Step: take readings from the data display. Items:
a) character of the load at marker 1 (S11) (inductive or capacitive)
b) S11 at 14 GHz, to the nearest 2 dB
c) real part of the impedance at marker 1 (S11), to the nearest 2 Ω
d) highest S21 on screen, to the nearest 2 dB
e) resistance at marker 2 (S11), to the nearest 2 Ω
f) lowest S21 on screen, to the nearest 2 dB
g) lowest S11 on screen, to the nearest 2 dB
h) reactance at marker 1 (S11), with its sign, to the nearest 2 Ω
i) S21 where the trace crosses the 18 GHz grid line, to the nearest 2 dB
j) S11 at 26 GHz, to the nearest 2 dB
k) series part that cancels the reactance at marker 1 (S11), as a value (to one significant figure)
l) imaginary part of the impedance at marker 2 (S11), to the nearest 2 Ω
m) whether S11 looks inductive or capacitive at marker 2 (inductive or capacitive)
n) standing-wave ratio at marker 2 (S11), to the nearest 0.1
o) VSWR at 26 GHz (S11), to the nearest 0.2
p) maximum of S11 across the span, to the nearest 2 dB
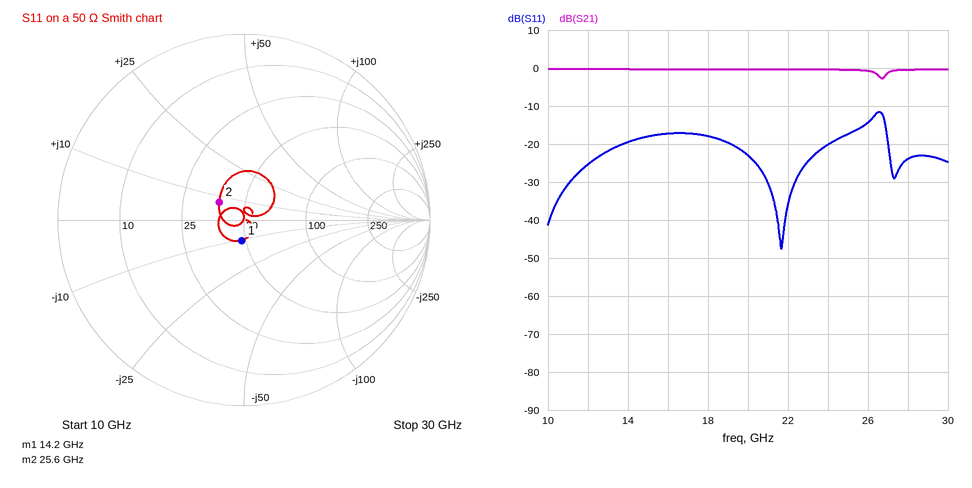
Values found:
capacitive
-20 dB
48 Ω
0 dB
38 Ω
-2 dB
-48 dB
-10 Ω
0 dB
-14 dB
100 pH
+8 Ω
inductive
1.4
1.4
-12 dB
